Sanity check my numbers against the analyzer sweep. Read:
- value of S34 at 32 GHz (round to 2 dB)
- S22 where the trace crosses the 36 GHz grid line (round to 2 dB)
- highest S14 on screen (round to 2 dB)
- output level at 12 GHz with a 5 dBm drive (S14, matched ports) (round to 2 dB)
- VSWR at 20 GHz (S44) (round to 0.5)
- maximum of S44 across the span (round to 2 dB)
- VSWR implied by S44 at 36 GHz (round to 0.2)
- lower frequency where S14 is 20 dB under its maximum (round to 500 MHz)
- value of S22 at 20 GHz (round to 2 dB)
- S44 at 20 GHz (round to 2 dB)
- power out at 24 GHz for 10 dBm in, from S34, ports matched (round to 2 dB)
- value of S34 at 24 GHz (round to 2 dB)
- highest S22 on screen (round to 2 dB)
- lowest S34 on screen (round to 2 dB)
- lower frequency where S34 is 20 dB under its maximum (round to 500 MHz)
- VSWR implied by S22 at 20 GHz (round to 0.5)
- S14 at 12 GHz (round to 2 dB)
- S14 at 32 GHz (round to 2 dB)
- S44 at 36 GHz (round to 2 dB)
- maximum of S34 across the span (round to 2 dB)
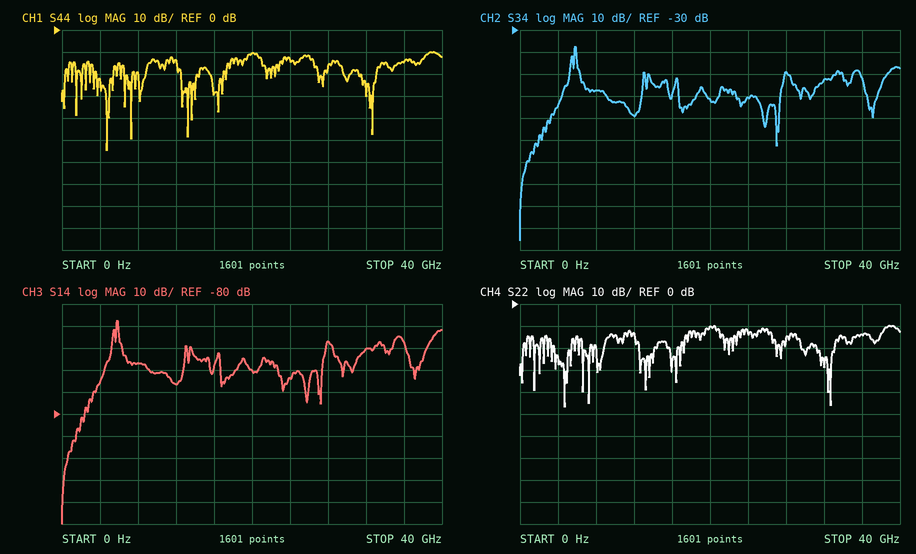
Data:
-52 dB
-14 dB
-38 dB
-62 dBm
2.0
-10 dB
1.4
4.5 GHz
-10 dB
-10 dB
-50 dBm
-60 dB
-10 dB
-126 dB
4.5 GHz
2.0
-66 dB
-50 dB
-14 dB
-38 dB
